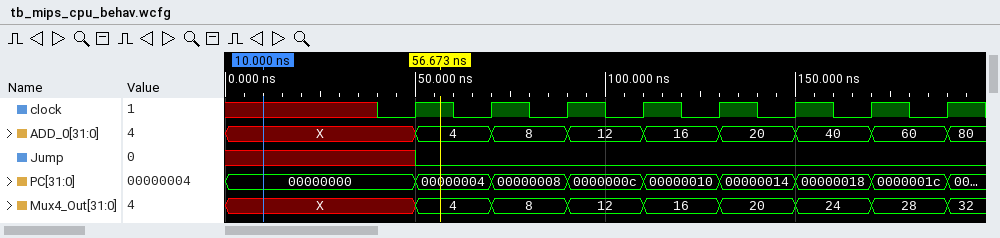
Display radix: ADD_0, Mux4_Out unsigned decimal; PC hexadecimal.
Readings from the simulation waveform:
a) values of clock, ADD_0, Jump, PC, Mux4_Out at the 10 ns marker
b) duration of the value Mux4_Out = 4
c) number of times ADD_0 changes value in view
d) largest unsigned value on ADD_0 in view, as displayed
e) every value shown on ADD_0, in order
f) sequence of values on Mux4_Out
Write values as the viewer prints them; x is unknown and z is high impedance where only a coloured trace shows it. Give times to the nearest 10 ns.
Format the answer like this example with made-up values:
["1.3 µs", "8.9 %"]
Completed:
["clock=x, ADD_0=X, Jump=x, PC=00000000, Mux4_Out=X", "20 ns", "8", "80", "X, 4, 8, 12, 16, 20, 40, 60, 80", "X, 4, 8, 12, 16, 20, 24, 28, 32"]
